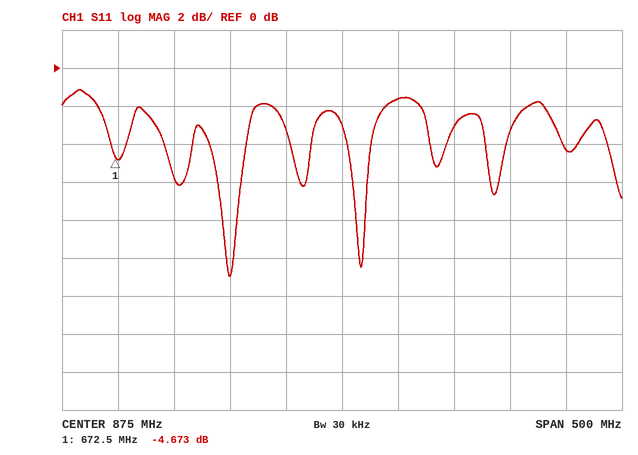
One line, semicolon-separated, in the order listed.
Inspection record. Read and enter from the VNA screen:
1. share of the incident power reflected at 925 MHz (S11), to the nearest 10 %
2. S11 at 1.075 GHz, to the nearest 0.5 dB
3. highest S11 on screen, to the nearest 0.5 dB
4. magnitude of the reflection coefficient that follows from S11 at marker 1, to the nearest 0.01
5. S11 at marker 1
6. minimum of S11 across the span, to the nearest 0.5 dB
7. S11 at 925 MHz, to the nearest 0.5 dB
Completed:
70 %; -4.5 dB; -1.0 dB; 0.58; -4.673 dB; -11.0 dB; -1.5 dB
